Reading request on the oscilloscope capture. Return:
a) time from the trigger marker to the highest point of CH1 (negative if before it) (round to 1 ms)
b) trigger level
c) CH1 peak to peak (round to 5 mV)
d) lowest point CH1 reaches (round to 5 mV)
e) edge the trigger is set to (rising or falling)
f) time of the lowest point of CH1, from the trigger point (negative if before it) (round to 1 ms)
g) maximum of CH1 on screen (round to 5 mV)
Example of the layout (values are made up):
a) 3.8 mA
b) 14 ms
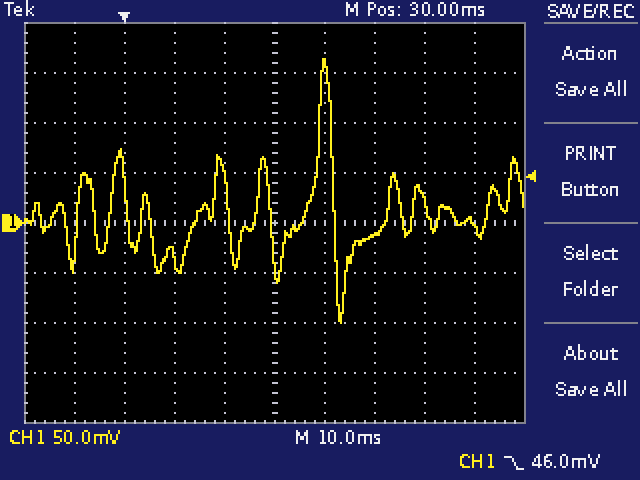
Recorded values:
a) +40 ms
b) 46.0 mV
c) 265 mV
d) -100 mV
e) falling
f) +43 ms
g) 165 mV
